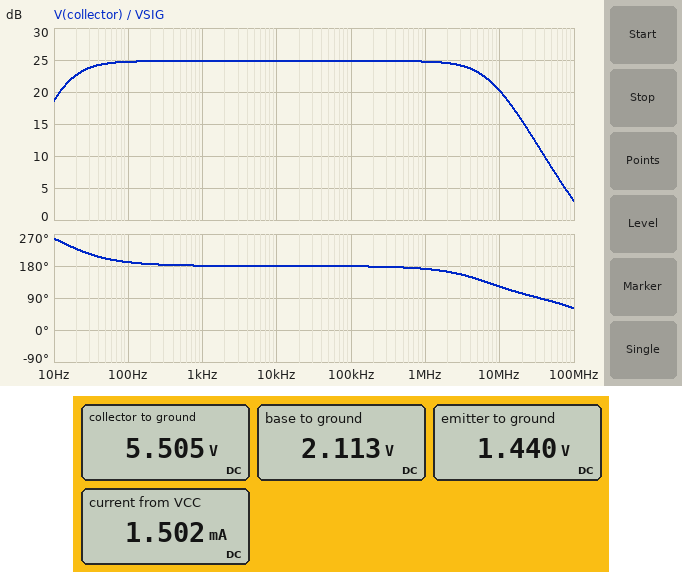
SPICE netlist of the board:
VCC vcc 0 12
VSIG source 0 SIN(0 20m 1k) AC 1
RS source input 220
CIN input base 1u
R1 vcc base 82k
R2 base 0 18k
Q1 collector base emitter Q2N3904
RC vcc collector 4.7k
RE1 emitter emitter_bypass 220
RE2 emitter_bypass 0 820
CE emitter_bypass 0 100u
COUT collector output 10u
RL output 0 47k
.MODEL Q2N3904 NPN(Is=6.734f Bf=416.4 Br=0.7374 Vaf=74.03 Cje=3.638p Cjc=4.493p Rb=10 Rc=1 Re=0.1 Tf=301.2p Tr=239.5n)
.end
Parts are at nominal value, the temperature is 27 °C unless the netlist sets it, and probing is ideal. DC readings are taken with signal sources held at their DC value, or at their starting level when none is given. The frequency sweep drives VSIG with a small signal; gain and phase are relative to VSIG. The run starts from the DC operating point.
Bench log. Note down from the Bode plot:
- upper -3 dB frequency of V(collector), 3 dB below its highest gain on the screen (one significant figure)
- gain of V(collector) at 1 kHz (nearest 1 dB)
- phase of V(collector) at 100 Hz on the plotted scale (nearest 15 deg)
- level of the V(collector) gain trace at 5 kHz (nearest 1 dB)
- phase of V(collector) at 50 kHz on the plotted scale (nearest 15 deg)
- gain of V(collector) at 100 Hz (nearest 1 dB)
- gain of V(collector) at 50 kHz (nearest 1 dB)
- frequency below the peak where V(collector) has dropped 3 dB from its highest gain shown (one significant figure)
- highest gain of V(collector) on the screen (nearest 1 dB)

7 MHz
25 dB
195 deg
25 dB
180 deg
25 dB
25 dB
20 Hz
25 dB
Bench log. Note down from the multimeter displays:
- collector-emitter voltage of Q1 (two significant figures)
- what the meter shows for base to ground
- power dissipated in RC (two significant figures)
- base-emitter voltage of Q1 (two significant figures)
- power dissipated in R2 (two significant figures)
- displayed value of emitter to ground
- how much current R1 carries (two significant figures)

4.1 V
2.113 V
9.0 mW
670 mV
250 µW
1.440 V
120 µA
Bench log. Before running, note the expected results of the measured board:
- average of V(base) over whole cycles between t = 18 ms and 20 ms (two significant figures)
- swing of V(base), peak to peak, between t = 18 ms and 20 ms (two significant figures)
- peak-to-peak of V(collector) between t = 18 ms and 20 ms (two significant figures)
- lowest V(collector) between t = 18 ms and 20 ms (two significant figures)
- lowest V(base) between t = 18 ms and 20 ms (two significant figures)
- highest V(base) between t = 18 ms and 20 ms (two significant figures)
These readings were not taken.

2.1 V
39 mV
700 mV
5.2 V
2.1 V
2.1 V
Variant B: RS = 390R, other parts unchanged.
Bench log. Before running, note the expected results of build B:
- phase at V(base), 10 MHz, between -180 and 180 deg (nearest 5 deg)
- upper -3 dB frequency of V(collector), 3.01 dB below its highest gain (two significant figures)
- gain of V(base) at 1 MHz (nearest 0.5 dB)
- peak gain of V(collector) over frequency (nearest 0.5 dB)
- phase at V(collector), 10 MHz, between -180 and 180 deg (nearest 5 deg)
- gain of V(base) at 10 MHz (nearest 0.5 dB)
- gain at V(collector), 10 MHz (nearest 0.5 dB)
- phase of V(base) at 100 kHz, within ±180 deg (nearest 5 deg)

-25 deg
5.3 MHz
-0.5 dB
24.5 dB
115 deg
-5.0 dB
18.0 dB
0 deg
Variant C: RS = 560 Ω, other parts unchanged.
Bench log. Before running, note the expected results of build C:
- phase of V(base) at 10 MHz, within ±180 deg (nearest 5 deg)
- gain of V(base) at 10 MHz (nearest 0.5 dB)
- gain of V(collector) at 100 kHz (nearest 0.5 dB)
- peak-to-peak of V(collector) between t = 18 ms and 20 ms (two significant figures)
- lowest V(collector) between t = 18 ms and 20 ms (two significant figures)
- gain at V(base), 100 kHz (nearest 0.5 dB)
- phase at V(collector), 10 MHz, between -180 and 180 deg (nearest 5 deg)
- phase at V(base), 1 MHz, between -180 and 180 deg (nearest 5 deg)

-30 deg
-7.0 dB
24.5 dB
680 mV
5.2 V
-0.5 dB
110 deg
-10 deg
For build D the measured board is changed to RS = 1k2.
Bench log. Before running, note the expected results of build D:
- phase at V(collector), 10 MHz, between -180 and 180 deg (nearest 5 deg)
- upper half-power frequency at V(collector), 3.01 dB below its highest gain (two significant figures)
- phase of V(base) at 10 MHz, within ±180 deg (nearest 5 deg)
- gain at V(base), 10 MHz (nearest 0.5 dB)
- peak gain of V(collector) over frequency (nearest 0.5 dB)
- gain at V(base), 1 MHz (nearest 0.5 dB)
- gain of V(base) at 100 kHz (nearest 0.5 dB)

100 deg
2.4 MHz
-40 deg
-11.5 dB
24.0 dB
-1.5 dB
-1.0 dB
